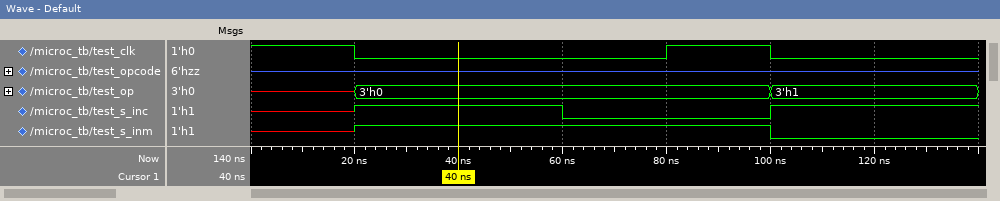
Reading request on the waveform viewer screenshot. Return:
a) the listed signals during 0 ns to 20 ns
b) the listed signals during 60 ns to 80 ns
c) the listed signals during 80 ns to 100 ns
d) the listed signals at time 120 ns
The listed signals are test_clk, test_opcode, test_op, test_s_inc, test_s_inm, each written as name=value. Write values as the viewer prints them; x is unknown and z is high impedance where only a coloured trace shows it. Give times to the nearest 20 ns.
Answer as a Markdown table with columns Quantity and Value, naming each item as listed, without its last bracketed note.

| Quantity | Value |
|---|---|
| the listed signals during 0 ns to 20 ns | test_clk=1, test_opcode=z, test_op=x, test_s_inc=x, test_s_inm=x |
| the listed signals during 60 ns to 80 ns | test_clk=0, test_opcode=z, test_op=3'h0, test_s_inc=0, test_s_inm=1 |
| the listed signals during 80 ns to 100 ns | test_clk=1, test_opcode=z, test_op=3'h0, test_s_inc=0, test_s_inm=1 |
| the listed signals at time 120 ns | test_clk=0, test_opcode=z, test_op=3'h1, test_s_inc=1, test_s_inm=0 |
